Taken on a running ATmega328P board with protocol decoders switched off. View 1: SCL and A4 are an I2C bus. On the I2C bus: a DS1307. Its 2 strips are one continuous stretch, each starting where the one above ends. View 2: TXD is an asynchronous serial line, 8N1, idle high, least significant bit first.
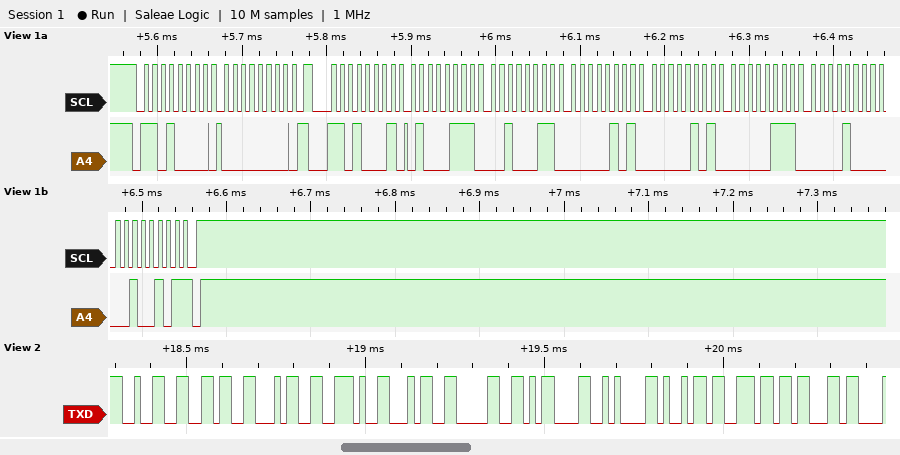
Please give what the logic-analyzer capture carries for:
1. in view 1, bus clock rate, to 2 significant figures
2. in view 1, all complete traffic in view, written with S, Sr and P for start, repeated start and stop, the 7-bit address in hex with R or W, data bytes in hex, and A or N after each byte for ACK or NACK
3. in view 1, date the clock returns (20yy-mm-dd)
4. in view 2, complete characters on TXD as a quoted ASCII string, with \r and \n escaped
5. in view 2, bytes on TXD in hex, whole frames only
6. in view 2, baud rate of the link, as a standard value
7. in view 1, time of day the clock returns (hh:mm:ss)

100 kHz
S 68W A 00 A Sr 68R A 47 A 23 A 05 A 05 A 07 A 08 A 25 N P
2025-08-07
"264.40\r\ninc"
32 36 34 2E 34 30 0D 0A 69 6E 63
57600 baud
05:23:47
